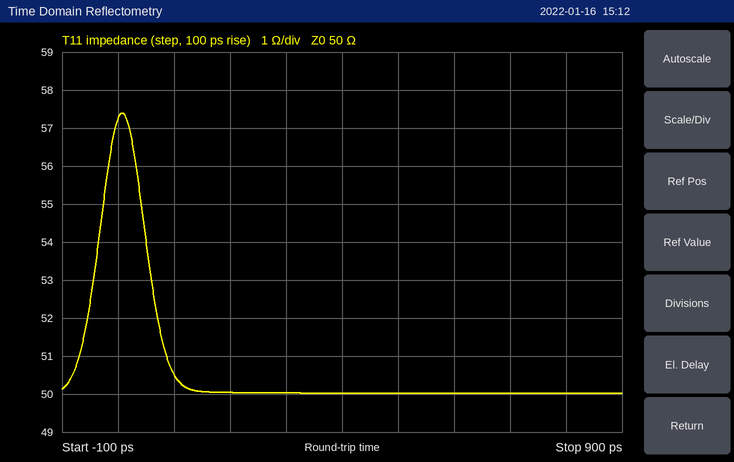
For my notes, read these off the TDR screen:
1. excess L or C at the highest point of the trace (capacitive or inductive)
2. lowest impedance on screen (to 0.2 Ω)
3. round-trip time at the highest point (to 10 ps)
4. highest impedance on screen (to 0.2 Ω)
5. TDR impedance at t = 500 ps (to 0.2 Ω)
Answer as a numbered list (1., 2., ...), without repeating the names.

1. inductive
2. 50.0 Ω
3. 10 ps
4. 57.4 Ω
5. 50.0 Ω
